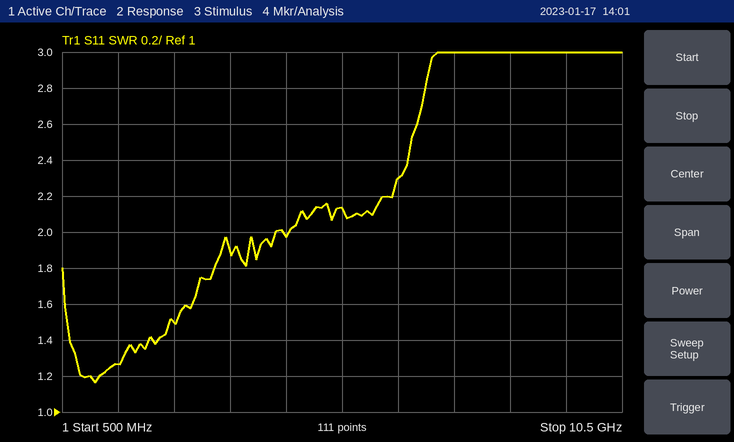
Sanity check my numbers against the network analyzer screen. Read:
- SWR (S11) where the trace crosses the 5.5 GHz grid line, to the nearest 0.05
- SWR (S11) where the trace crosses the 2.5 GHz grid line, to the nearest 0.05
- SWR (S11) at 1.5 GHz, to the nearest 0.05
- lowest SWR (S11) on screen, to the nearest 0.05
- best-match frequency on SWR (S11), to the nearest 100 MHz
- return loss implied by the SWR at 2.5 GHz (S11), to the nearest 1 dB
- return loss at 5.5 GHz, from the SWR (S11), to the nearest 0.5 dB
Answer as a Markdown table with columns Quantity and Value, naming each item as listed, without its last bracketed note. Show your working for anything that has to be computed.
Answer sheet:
| Quantity | Value |
|---|---|
| SWR (S11) where the trace crosses the 5.5 GHz grid line, to the nearest 0.05 | 2.15 |
| SWR (S11) where the trace crosses the 2.5 GHz grid line, to the nearest 0.05 | 1.50 |
| SWR (S11) at 1.5 GHz, to the nearest 0.05 | 1.25 |
| lowest SWR (S11) on screen, to the nearest 0.05 | 1.15 |
| best-match frequency on SWR (S11), to the nearest 100 MHz | 1.1 GHz |
| return loss implied by the SWR at 2.5 GHz (S11), to the nearest 1 dB | −20 log10((1.5 − 1)/(1.5 + 1)) ≈ 14 dB |
| return loss at 5.5 GHz, from the SWR (S11), to the nearest 0.5 dB | −20 log10((2.15 − 1)/(2.15 + 1)) ≈ 8.75 dB, so 9.0 dB to the nearest 0.5 dB |
